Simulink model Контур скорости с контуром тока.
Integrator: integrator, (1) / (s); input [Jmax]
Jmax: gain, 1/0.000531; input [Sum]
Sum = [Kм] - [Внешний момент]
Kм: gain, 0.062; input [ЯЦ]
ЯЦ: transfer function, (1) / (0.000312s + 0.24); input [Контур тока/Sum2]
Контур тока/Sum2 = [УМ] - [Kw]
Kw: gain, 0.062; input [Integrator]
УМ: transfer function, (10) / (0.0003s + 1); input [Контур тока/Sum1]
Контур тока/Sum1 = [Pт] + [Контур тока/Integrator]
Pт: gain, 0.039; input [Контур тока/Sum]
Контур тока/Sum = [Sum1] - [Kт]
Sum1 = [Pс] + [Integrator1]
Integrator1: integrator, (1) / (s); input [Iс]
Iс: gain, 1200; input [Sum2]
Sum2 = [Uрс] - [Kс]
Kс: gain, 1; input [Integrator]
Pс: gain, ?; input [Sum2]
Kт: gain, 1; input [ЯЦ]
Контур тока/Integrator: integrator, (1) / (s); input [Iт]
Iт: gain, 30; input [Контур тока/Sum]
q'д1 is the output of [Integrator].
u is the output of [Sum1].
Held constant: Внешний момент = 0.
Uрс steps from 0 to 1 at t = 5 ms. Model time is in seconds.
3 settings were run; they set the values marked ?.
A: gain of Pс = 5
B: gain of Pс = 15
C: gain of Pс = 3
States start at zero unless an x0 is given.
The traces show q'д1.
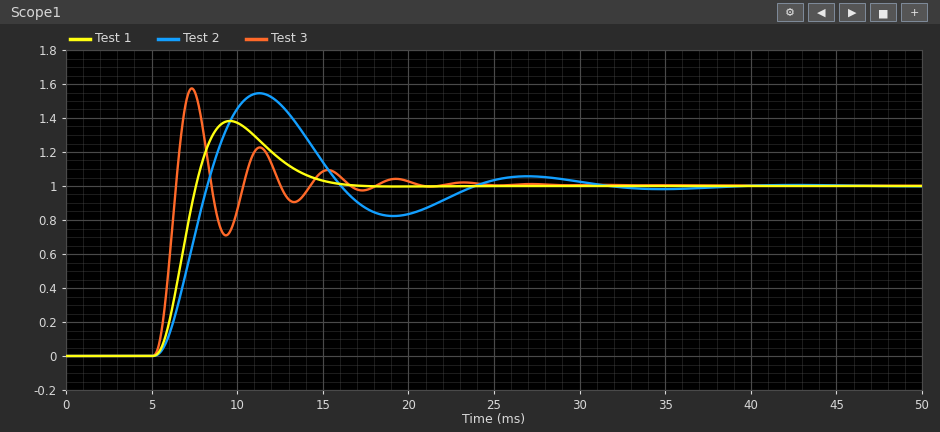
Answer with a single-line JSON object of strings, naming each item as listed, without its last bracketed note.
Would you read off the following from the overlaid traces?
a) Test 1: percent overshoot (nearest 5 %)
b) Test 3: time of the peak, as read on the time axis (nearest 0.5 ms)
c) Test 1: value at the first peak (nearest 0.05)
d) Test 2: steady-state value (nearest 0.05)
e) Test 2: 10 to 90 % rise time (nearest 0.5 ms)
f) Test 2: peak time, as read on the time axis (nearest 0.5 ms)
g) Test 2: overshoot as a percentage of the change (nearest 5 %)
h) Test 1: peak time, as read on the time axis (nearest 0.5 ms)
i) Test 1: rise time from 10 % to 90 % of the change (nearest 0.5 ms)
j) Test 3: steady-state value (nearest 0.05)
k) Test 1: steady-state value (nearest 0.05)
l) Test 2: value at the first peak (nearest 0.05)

{"Test 1: percent overshoot": "40 %", "Test 3: time of the peak, as read on the time axis": "7.5 ms", "Test 1: value at the first peak": "1.40", "Test 2: steady-state value": "1.00", "Test 2: 10 to 90 % rise time": "2.0 ms", "Test 2: peak time, as read on the time axis": "11.5 ms", "Test 2: overshoot as a percentage of the change": "55 %", "Test 1: peak time, as read on the time axis": "9.5 ms", "Test 1: rise time from 10 % to 90 % of the change": "1.5 ms", "Test 3: steady-state value": "1.00", "Test 1: steady-state value": "1.00", "Test 2: value at the first peak": "1.55"}
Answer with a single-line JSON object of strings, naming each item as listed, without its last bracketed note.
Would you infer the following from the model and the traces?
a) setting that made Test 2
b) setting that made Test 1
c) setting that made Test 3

{"setting that made Test 2": "C", "setting that made Test 1": "A", "setting that made Test 3": "B"}
